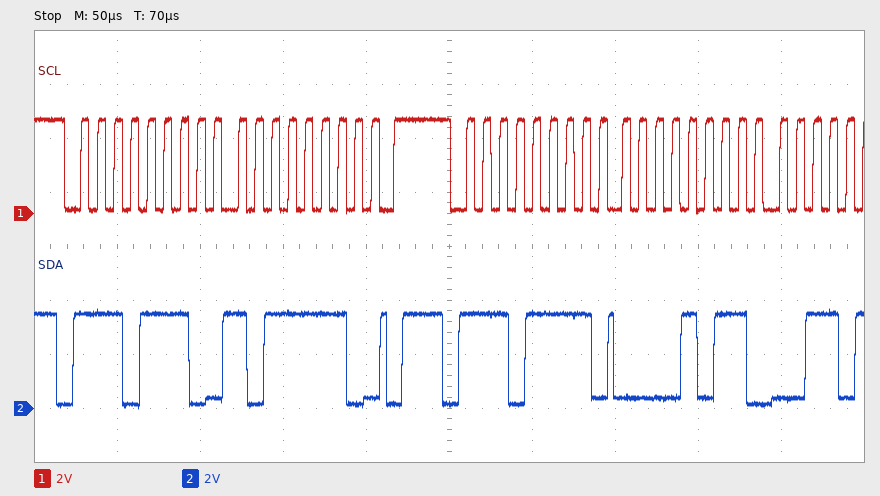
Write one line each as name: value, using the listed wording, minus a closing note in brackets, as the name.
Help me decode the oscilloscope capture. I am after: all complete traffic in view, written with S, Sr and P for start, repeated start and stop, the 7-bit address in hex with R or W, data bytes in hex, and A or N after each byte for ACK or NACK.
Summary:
all complete traffic in view, written with S, Sr and P for start, repeated start and stop, the 7-bit address in hex with R or W, data bytes in hex, and A or N after each byte for ACK or NACK: S 77W A BE A P S 77R A 0B A
